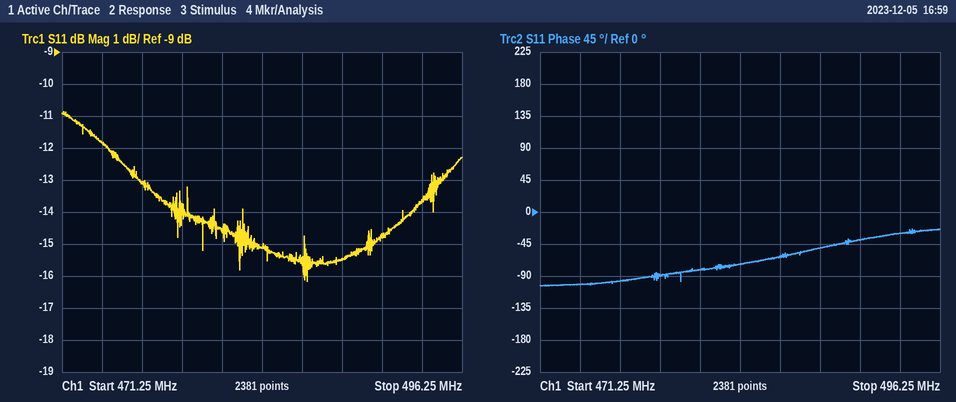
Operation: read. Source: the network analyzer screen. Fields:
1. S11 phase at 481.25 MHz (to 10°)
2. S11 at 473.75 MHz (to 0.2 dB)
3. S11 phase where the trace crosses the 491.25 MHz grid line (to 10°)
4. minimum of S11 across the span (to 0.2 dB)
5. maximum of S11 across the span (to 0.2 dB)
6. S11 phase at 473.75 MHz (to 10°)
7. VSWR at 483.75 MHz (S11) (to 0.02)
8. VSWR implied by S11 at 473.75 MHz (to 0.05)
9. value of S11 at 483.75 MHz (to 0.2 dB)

-80°
-11.8 dB
-40°
-16.2 dB
-10.8 dB
-100°
1.42
1.70
-15.2 dB
